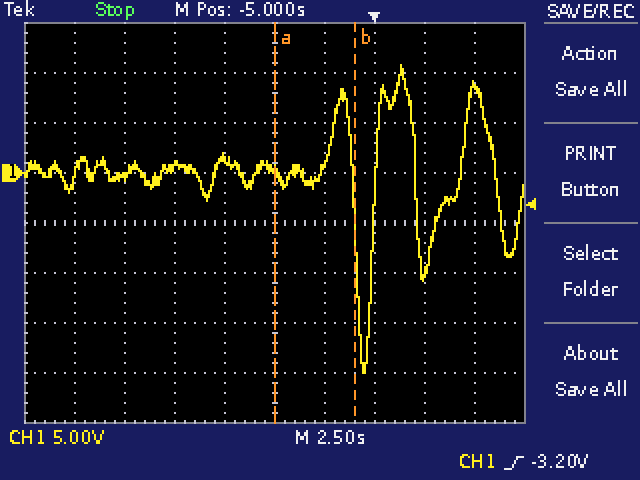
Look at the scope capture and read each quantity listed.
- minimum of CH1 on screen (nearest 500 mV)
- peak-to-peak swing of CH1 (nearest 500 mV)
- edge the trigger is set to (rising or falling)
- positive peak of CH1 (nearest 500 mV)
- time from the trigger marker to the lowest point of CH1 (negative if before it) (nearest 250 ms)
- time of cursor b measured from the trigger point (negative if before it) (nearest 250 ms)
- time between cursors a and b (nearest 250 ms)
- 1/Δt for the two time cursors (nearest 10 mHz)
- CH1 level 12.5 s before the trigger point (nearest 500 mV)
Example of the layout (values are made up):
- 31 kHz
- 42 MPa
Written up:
- -20.0 V
- 31.0 V
- rising
- 11.0 V
- -500 ms
- -1.00 s
- 4.00 s
- 250 mHz
- -500 mV
